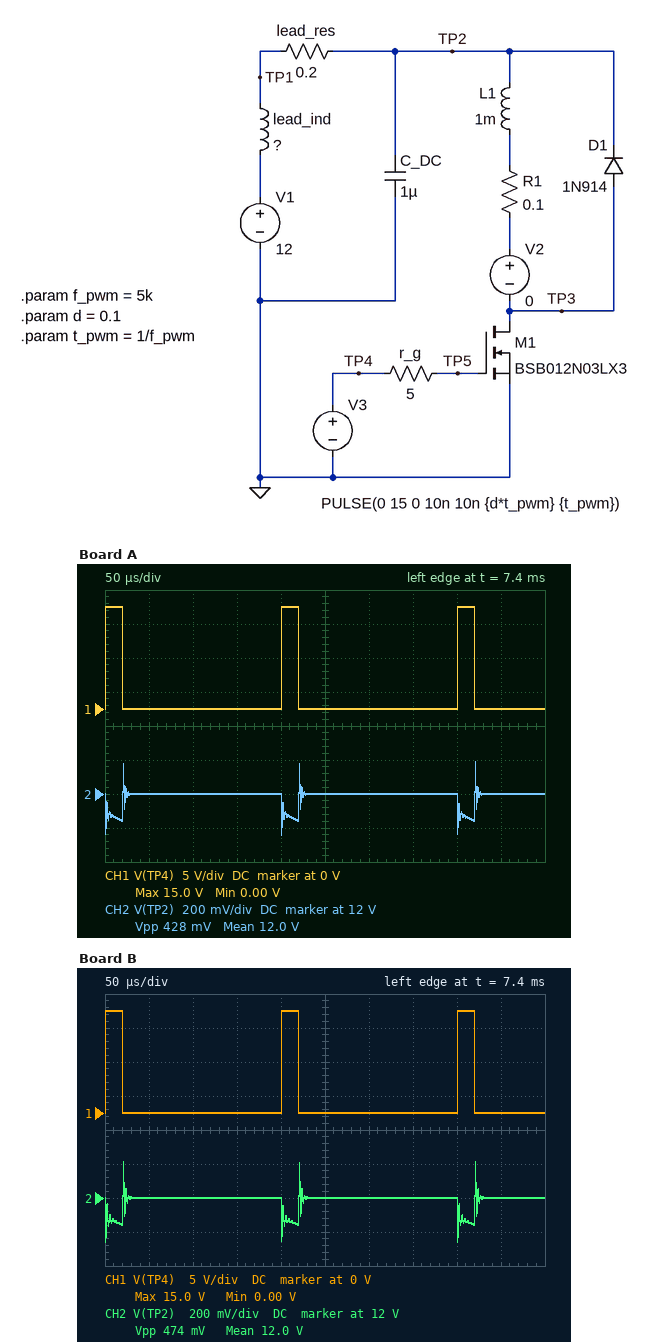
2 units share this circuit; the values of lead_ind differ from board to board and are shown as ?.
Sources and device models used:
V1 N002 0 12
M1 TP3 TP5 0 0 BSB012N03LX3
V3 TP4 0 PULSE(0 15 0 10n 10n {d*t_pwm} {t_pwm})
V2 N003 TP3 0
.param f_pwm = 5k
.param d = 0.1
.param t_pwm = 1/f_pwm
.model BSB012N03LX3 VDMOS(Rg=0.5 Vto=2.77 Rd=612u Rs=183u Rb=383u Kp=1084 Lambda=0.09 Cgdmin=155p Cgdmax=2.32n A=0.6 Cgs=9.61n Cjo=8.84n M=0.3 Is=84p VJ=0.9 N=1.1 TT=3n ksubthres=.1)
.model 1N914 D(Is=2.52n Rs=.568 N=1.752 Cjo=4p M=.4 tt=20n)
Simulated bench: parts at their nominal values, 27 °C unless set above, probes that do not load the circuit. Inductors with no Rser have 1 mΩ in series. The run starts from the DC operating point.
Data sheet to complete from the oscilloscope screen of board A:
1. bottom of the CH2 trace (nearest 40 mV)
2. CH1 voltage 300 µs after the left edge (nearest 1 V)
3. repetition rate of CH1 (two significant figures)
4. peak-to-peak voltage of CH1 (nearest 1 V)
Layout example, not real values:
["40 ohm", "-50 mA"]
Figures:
["11.76 V", "0 V", "5.0 kHz", "15 V"]
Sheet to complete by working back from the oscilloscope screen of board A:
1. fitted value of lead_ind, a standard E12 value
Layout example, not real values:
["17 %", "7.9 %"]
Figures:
["150 nH"]
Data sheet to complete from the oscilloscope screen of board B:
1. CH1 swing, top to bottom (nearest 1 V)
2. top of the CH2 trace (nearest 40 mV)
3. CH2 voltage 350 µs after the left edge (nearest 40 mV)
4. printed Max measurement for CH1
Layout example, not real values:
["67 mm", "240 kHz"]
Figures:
["15 V", "12.20 V", "12.00 V", "15.0 V"]
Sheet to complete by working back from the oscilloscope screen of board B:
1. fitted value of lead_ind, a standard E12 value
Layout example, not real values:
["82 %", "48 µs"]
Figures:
["180 nH"]
